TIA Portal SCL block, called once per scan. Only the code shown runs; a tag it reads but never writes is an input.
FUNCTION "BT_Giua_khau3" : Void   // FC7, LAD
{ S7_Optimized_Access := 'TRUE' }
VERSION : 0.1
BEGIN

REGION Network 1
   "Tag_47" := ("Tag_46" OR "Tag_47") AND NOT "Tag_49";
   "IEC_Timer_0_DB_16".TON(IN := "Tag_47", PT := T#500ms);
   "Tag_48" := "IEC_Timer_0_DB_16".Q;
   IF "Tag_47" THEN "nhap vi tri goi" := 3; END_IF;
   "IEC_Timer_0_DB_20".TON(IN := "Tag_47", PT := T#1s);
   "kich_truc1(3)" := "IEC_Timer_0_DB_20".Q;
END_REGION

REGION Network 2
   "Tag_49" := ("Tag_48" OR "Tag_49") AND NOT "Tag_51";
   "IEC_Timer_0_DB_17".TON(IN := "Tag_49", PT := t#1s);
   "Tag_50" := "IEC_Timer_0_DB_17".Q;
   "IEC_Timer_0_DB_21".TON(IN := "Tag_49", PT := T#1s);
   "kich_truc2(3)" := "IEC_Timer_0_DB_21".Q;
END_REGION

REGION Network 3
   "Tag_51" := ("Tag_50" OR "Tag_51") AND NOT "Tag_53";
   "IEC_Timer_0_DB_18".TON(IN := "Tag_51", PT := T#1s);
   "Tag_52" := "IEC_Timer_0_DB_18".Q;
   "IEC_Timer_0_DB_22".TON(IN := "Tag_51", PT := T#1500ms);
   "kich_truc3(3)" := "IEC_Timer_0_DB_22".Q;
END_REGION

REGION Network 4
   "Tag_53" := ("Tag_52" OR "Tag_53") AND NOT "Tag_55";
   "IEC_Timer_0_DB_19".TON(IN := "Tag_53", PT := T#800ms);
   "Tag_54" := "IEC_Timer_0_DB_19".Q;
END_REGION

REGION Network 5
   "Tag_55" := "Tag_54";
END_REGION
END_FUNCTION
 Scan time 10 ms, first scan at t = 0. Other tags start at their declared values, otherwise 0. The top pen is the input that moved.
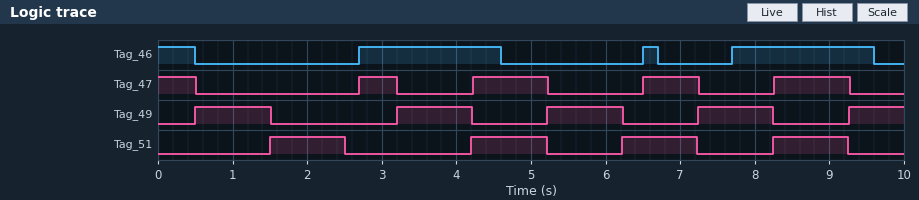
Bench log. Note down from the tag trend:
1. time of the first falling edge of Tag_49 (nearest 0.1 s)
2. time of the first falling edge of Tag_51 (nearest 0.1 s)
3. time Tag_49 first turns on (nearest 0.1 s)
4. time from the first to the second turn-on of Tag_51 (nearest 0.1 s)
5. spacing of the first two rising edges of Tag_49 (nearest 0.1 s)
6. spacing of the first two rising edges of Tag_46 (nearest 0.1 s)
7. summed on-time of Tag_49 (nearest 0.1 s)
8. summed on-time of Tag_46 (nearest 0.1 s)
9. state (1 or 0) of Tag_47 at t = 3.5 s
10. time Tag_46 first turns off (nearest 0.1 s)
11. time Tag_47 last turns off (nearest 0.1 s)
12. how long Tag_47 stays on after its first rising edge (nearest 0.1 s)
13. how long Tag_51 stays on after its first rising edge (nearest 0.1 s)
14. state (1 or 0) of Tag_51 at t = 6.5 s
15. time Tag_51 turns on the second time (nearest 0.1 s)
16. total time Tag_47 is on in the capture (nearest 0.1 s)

1.5 s
2.5 s
0.5 s
2.7 s
2.7 s
3.8 s
4.8 s
4.5 s
0
0.5 s
9.3 s
0.5 s
1.0 s
1
4.2 s
3.8 s
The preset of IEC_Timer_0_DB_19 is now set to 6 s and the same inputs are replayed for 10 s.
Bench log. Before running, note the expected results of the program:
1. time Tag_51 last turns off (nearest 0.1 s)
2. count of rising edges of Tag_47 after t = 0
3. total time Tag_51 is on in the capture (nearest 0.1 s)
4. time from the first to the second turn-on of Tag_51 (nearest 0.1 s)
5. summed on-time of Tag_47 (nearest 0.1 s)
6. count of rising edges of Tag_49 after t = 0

9.5 s
2
2.0 s
7.0 s
2.0 s
3
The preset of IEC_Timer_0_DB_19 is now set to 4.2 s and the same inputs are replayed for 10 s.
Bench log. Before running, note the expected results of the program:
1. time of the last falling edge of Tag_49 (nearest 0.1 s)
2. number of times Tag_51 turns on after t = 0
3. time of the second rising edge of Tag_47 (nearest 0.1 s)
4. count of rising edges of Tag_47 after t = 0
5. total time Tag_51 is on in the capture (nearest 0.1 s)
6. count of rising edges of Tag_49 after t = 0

6.7 s
2
7.7 s
2
2.0 s
3
